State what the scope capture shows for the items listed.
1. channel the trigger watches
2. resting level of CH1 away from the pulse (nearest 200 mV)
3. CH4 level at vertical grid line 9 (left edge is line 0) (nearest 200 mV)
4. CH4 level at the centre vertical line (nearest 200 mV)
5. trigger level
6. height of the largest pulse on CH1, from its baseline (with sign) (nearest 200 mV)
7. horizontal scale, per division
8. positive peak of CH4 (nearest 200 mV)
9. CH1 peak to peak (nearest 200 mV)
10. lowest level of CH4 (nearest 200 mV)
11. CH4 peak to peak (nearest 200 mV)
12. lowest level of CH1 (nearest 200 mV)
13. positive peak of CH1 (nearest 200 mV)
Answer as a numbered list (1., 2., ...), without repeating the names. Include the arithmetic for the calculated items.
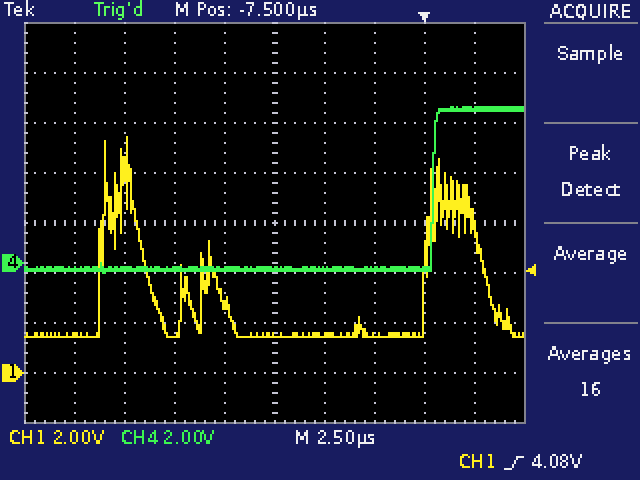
1. CH1
2. 1.4 V
3. 6.2 V
4. -200 mV
5. 4.08 V
6. 9.4 V − (1.4 V) = +8.0 V
7. 2.5 µs
8. 6.2 V
9. 9.4 V − (1.4 V) = 8.0 V
10. -400 mV
11. 6.2 V − (-400 mV) = 6.6 V
12. 1.4 V
13. 9.4 V
